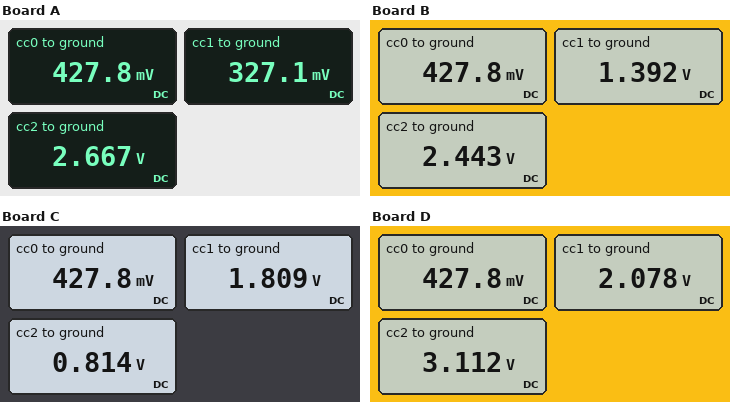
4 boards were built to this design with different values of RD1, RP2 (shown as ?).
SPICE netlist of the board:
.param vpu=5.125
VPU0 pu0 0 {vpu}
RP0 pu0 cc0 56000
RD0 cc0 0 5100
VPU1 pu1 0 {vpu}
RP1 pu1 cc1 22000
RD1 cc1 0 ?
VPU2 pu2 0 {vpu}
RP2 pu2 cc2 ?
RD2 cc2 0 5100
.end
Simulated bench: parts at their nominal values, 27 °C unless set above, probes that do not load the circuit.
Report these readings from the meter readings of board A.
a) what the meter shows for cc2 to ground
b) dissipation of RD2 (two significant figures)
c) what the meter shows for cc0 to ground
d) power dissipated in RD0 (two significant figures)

2.667 V
1.4 mW
427.8 mV
36 µW
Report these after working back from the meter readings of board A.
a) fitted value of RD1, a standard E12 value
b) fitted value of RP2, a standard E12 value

1.5 kΩ
4.7 kΩ
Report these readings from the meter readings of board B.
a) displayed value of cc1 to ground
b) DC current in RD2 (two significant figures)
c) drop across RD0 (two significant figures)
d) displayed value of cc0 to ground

1.392 V
480 µA
430 mV
427.8 mV
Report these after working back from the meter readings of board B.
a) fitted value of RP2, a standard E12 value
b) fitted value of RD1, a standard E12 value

5.6 kΩ
8.2 kΩ
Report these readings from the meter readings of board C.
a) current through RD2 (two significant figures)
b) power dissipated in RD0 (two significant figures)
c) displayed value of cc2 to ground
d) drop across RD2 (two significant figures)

160 µA
36 µW
0.814 V
810 mV
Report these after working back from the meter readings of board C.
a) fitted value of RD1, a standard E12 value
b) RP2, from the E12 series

12 kΩ
27 kΩ
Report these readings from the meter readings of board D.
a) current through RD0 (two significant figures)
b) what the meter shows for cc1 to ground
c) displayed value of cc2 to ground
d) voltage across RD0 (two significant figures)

84 µA
2.078 V
3.112 V
430 mV
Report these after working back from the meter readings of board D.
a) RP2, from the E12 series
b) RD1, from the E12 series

3.3 kΩ
15 kΩ
